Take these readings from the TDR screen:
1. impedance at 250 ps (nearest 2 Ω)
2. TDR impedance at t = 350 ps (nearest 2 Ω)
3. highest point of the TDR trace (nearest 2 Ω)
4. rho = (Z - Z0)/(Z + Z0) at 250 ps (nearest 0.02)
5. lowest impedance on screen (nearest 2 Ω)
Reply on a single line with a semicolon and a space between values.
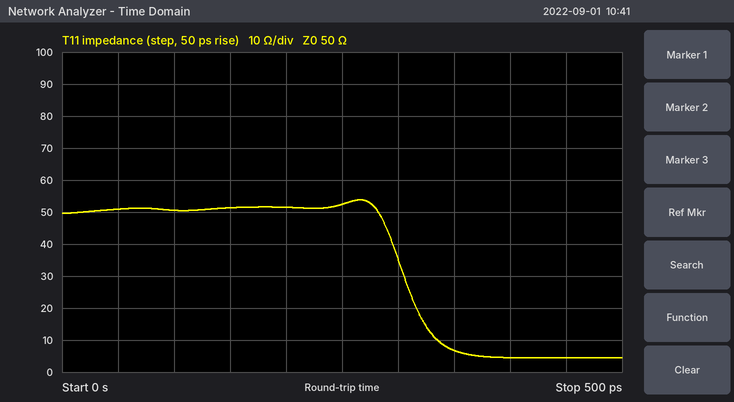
52 Ω; 6 Ω; 54 Ω; +0.02; 4 Ω
